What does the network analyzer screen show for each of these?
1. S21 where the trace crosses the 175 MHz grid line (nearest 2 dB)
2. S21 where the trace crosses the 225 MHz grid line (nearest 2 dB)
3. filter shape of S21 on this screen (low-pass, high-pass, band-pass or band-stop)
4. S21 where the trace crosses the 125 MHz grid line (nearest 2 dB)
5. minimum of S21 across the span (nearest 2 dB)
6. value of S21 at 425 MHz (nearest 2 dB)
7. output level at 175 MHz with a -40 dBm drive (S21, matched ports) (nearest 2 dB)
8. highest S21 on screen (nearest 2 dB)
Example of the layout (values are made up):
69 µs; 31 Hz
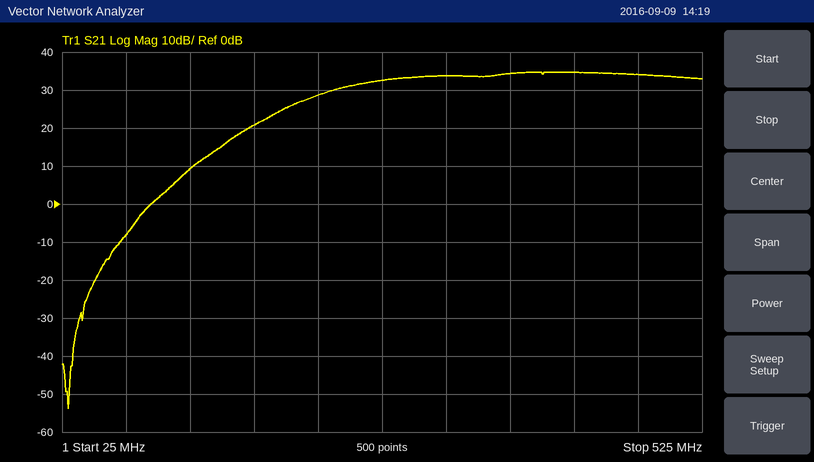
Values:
20 dB; 28 dB; high-pass; 10 dB; -54 dB; 34 dB; -20 dBm; 34 dB
